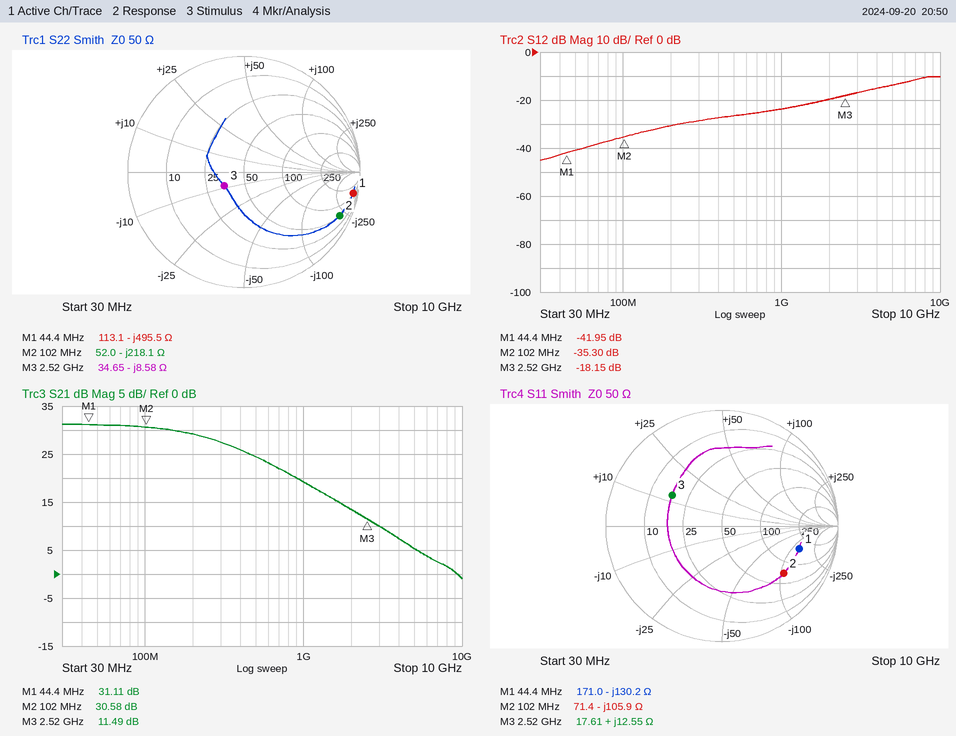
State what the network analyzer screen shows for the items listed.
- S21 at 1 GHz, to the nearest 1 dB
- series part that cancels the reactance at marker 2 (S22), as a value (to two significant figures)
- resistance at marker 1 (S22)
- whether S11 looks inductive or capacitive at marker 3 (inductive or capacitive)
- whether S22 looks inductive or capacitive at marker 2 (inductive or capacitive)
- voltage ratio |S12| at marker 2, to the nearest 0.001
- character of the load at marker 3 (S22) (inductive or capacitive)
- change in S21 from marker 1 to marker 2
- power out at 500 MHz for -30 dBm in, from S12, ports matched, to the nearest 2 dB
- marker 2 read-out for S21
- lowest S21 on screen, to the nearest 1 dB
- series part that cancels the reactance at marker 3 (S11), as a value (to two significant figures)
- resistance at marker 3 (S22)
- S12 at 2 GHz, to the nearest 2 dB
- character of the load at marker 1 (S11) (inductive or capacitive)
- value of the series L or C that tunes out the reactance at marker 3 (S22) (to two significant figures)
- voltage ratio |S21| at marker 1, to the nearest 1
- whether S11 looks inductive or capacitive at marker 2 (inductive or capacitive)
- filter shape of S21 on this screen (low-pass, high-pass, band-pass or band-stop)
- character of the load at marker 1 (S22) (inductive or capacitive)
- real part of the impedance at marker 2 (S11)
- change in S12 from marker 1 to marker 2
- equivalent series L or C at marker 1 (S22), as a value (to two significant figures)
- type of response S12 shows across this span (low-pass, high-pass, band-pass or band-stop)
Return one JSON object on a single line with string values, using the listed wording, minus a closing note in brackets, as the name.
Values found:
{"S21 at 1 GHz, to the nearest 1 dB": "19 dB", "series part that cancels the reactance at marker 2 (S22), as a value": "340 nH", "resistance at marker 1": "113.1 Ω", "whether S11 looks inductive or capacitive at marker 3": "inductive", "whether S22 looks inductive or capacitive at marker 2": "capacitive", "voltage ratio |S12| at marker 2, to the nearest 0.001": "0.017", "character of the load at marker 3 (S22)": "capacitive", "change in S21 from marker 1 to marker 2": "-0.53 dB", "power out at 500 MHz for -30 dBm in, from S12, ports matched, to the nearest 2 dB": "-56 dBm", "marker 2 read-out for S21": "30.58 dB", "lowest S21 on screen, to the nearest 1 dB": "-1 dB", "series part that cancels the reactance at marker 3 (S11), as a value": "5.0 pF", "resistance at marker 3": "34.65 Ω", "S12 at 2 GHz, to the nearest 2 dB": "-20 dB", "character of the load at marker 1 (S11)": "capacitive", "value of the series L or C that tunes out the reactance at marker 3 (S22)": "540 pH", "voltage ratio |S21| at marker 1, to the nearest 1": "36", "whether S11 looks inductive or capacitive at marker 2": "capacitive", "filter shape of S21 on this screen": "low-pass", "character of the load at marker 1 (S22)": "capacitive", "real part of the impedance at marker 2": "71.4 Ω", "change in S12 from marker 1 to marker 2": "6.65 dB", "equivalent series L or C at marker 1 (S22), as a value": "7.2 pF", "type of response S12 shows across this span": "high-pass"}
